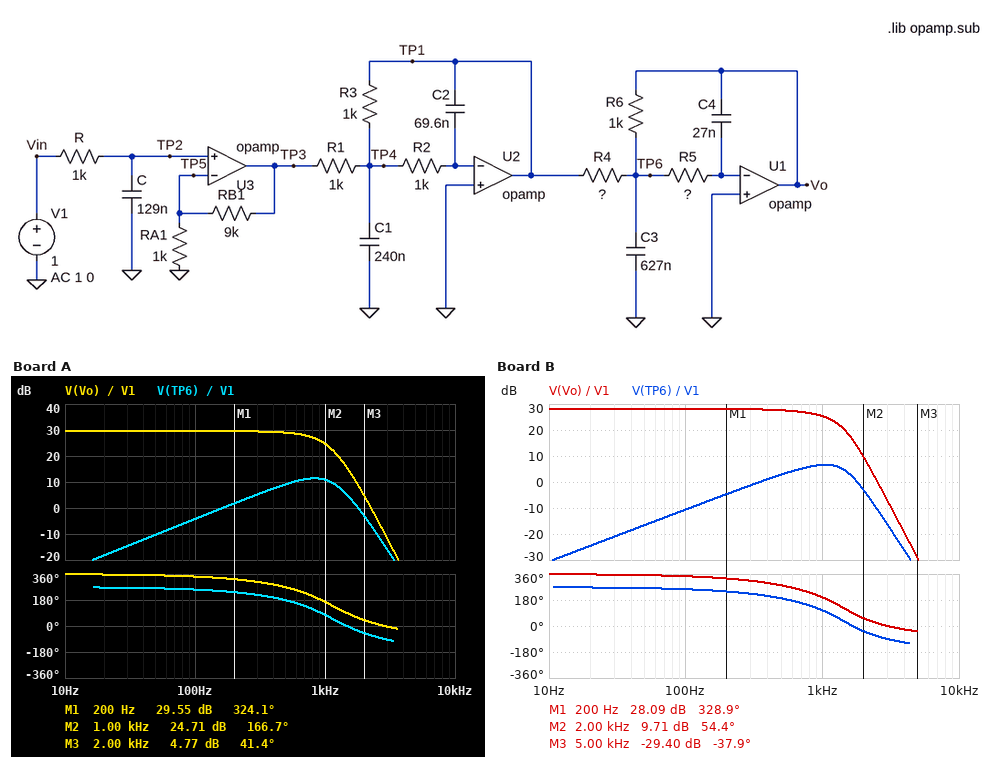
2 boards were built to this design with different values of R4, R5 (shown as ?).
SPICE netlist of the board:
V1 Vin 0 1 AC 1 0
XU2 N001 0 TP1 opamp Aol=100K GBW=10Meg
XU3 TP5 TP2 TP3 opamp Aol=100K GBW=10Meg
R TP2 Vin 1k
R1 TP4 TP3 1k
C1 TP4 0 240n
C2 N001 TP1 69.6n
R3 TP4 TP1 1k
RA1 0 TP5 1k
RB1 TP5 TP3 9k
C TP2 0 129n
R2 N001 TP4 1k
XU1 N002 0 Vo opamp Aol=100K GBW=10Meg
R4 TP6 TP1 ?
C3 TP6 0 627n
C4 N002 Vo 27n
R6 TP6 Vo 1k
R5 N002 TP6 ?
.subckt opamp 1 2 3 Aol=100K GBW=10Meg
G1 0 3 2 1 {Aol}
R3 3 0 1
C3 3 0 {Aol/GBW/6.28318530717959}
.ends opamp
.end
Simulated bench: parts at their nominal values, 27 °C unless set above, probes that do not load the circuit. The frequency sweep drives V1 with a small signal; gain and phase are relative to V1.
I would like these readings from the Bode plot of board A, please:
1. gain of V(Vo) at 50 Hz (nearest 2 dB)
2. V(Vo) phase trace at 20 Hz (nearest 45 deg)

30 dB
360 deg
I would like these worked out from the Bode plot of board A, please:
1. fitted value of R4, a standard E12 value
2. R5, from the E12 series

330 Ω
1.2 kΩ
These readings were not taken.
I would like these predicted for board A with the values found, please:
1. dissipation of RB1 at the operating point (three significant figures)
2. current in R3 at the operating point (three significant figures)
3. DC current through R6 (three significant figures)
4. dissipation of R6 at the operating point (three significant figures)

9.00 mW
10.0 mA
30.3 mA
918 mW
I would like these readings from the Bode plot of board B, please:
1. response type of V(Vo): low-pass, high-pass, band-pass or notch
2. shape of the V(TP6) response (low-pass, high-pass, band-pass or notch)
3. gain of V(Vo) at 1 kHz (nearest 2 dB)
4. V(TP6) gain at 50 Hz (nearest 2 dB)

low-pass
band-pass
26 dB
-16 dB
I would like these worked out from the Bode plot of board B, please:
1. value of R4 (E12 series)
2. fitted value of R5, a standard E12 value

390 Ω
680 Ω
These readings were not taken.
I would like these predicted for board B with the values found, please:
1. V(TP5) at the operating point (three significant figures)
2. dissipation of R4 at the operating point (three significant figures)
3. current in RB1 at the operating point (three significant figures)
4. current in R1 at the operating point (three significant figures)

1.00 V
256 mW
1.00 mA
10.0 mA
